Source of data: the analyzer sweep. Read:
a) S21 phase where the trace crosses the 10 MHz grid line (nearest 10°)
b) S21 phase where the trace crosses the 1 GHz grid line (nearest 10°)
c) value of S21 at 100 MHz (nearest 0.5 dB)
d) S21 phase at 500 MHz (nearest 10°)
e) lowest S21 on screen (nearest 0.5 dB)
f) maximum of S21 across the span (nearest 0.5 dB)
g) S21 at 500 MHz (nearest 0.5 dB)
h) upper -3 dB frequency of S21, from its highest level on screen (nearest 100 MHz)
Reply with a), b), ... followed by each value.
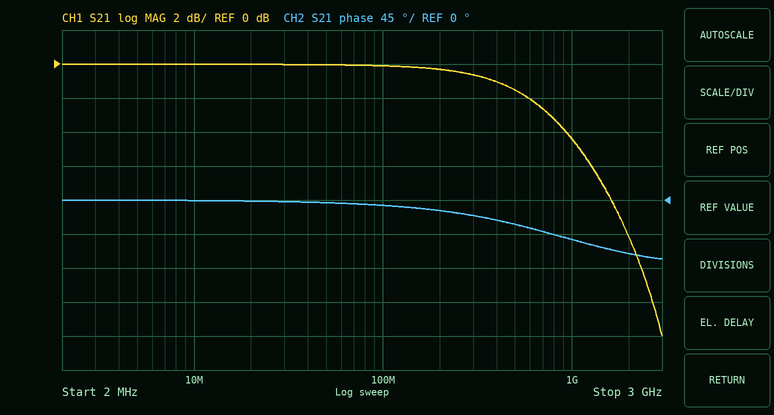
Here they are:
a) 0°
b) -50°
c) 0.0 dB
d) -30°
e) -16.0 dB
f) 0.0 dB
g) -1.5 dB
h) 800 MHz
